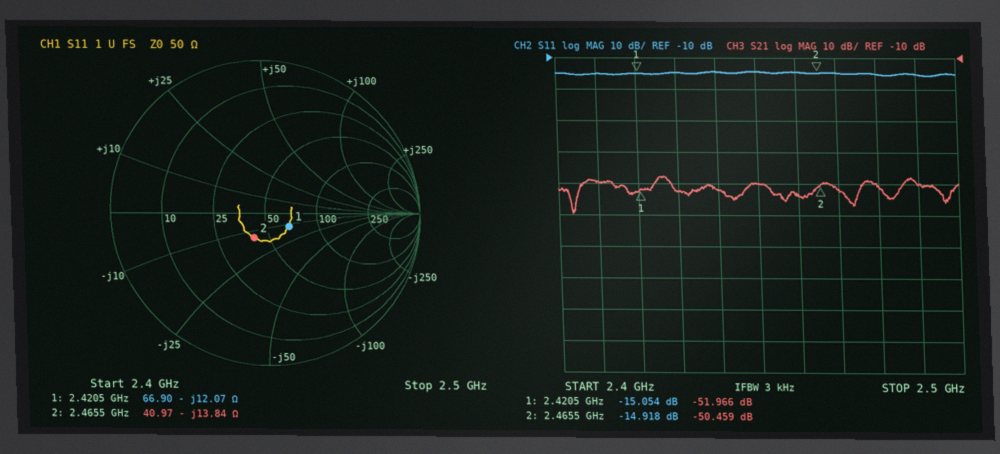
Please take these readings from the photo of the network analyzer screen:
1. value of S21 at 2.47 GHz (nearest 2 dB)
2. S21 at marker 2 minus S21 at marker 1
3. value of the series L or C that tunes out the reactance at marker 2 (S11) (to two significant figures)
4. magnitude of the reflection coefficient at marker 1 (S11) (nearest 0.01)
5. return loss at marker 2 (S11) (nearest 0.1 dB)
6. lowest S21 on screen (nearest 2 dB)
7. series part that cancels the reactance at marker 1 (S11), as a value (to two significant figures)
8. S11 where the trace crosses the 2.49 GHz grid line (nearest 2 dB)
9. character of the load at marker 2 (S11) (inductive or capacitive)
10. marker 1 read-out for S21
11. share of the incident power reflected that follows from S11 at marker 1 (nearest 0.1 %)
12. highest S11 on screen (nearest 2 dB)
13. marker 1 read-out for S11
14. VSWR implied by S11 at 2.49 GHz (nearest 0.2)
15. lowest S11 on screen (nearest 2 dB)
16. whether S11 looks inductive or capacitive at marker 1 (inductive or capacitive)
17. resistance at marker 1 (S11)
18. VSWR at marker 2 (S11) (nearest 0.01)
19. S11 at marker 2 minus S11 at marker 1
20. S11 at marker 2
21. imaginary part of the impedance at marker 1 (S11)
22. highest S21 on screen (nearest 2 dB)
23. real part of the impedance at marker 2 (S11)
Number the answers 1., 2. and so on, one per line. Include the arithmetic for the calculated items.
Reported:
1. -52 dB
2. -50.459 − (-51.966) = 1.507 dB
3. L = 13.84 Ω/(2π × 2.4655 GHz) ≈ 893 pH, so 890 pH to two significant figures
4. 0.18
5. 14.9 dB
6. -60 dB
7. L = 12.07 Ω/(2π × 2.4205 GHz) ≈ 794 pH, so 790 pH to two significant figures
8. -16 dB
9. capacitive
10. -51.966 dB
11. 10^(-15.054/10) ≈ 3.1 %
12. -14 dB
13. -15.054 dB
14. |Γ| = 10^(-16/20) = 0.1585; VSWR = (1 + 0.1585)/(1 − 0.1585) ≈ 1.4
15. -16 dB
16. capacitive
17. 66.90 Ω
18. (1 + 0.1795)/(1 − 0.1795) ≈ 1.44
19. -14.918 − (-15.054) = 0.136 dB
20. -14.918 dB
21. -12.07 Ω
22. -48 dB
23. 40.97 Ω
